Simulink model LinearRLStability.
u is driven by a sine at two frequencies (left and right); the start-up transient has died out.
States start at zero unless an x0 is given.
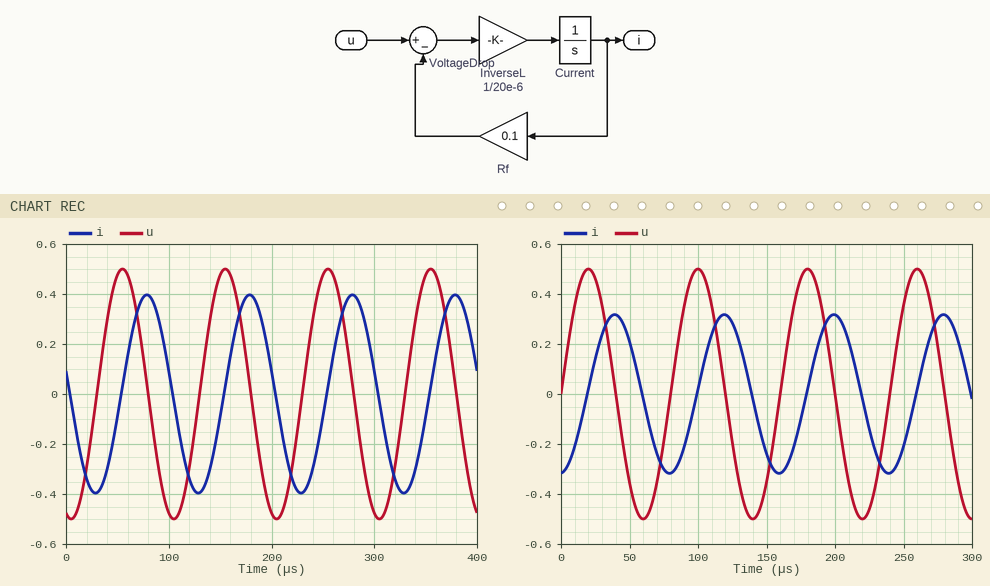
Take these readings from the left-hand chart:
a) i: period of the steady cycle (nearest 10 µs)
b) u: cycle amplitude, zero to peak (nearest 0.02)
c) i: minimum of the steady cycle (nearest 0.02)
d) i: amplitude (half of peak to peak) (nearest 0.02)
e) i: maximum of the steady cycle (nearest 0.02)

100 µs
0.50
-0.40
0.40
0.40
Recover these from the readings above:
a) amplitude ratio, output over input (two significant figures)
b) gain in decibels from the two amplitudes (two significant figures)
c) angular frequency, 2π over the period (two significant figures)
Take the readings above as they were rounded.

0.80
-1.9 dB
0.063 rad/µs
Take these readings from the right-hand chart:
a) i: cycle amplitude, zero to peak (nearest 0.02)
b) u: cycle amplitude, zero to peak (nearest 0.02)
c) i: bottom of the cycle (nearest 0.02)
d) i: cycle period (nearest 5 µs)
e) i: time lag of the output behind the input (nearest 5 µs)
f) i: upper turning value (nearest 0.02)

0.32
0.50
-0.32
80 µs
20 µs
0.32
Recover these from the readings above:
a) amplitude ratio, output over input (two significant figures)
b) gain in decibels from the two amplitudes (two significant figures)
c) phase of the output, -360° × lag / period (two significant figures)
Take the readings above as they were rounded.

0.64
-3.9 dB
-90°
